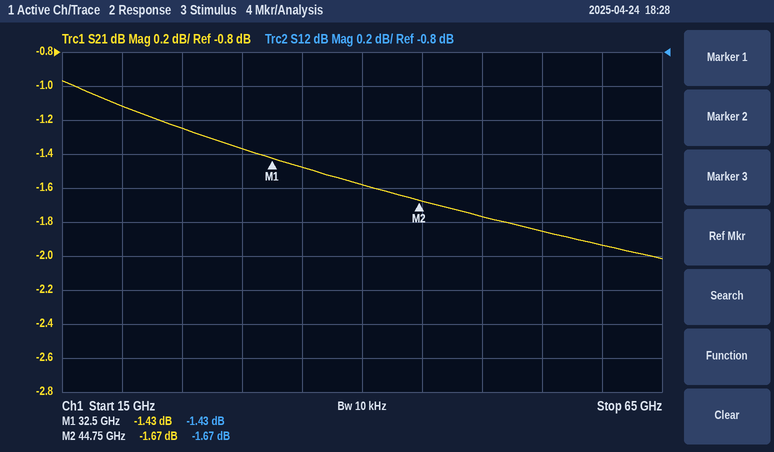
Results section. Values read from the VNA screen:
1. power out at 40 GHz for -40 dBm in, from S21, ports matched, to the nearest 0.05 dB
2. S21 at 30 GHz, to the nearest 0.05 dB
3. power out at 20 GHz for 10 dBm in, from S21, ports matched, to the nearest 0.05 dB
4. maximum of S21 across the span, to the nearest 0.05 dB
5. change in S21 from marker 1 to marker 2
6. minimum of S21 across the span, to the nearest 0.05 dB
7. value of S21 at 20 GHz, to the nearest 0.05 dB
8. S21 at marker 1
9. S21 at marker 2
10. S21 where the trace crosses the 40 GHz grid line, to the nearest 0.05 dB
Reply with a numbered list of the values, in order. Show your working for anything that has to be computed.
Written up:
1. -40 dBm + (-1.60 dB) = -41.60 dBm
2. -1.35 dB
3. 10 dBm + (-1.10 dB) = 8.90 dBm
4. -0.95 dB
5. -1.67 − (-1.43) = -0.24 dB
6. -2.00 dB
7. -1.10 dB
8. -1.43 dB
9. -1.67 dB
10. -1.60 dB
